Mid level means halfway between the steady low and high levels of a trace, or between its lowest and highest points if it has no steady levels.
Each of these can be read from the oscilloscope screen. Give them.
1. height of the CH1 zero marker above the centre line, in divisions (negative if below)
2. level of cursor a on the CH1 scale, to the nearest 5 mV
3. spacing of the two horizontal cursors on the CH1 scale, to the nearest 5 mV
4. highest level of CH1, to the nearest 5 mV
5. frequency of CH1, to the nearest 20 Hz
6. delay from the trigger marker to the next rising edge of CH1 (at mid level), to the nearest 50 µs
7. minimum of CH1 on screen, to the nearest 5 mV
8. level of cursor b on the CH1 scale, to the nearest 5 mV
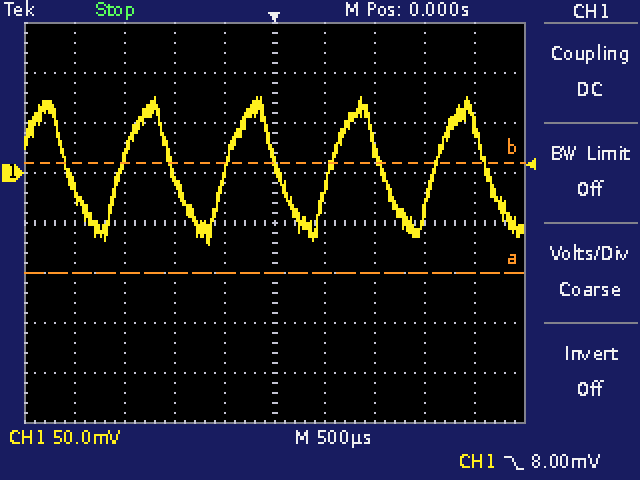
+1.0 div
-100 mV
110 mV
75 mV
960 Hz
550 µs
-70 mV
10 mV
